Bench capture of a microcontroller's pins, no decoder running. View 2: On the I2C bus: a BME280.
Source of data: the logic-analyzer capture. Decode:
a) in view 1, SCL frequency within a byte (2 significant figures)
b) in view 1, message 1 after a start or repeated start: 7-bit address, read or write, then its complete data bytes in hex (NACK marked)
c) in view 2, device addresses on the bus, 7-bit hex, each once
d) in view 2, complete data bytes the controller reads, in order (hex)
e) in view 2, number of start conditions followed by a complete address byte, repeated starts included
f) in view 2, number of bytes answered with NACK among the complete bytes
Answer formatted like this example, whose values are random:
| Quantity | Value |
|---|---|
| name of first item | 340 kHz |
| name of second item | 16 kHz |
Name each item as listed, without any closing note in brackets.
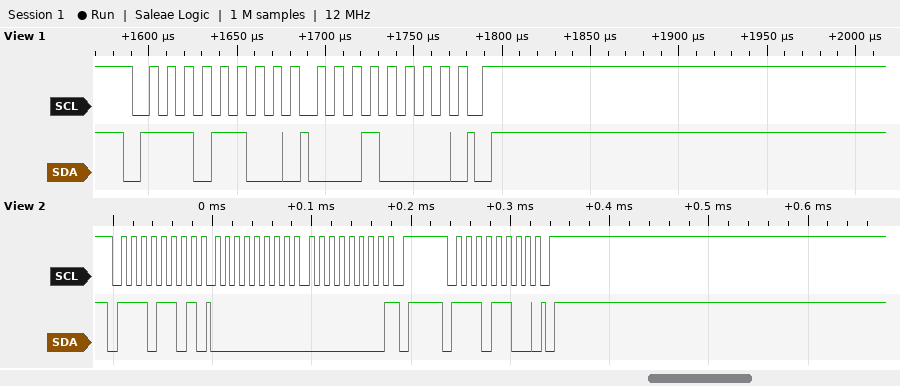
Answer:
| Quantity | Value |
|---|---|
| in view 1, SCL frequency within a byte | 100 kHz |
| in view 1, message 1 after a start or repeated start: 7-bit address, read or write, then its complete data bytes in hex | 0x76 write: 10 |
| in view 2, device addresses on the bus, 7-bit hex, each once | 0x76 |
| in view 2, complete data bytes the controller reads, in order | 00 00 |
| in view 2, number of start conditions followed by a complete address byte, repeated starts included | 2 |
| in view 2, number of bytes answered with NACK among the complete bytes | 1 |
